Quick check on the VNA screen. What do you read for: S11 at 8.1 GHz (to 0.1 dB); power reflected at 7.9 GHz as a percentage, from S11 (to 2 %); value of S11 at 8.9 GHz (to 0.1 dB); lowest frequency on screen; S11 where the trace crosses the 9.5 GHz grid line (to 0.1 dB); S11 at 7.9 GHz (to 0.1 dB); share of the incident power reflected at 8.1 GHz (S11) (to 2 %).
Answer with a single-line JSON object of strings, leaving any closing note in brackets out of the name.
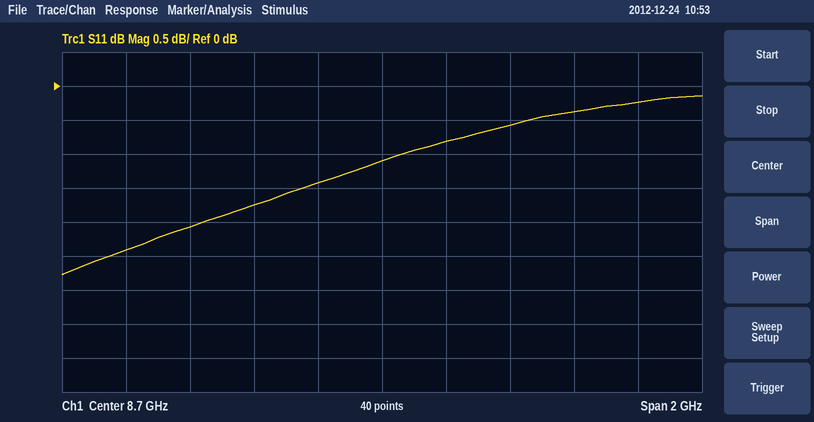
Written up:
{"S11 at 8.1 GHz": "-2.1 dB", "power reflected at 7.9 GHz as a percentage, from S11": "58 %", "value of S11 at 8.9 GHz": "-0.8 dB", "lowest frequency on screen": "7.7 GHz", "S11 where the trace crosses the 9.5 GHz grid line": "-0.2 dB", "S11 at 7.9 GHz": "-2.4 dB", "share of the incident power reflected at 8.1 GHz (S11)": "62 %"}
